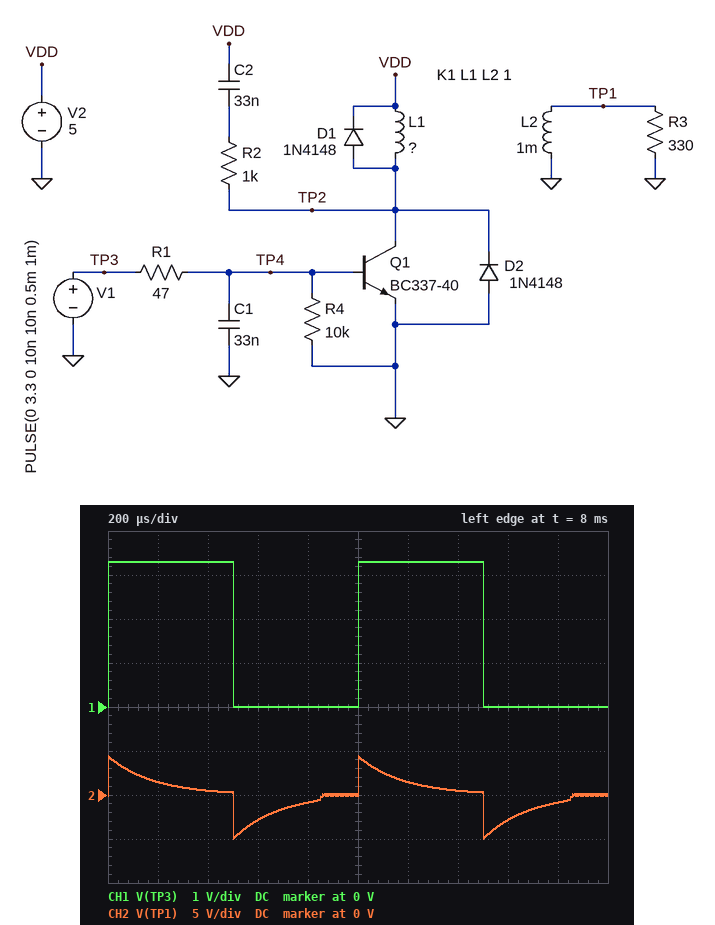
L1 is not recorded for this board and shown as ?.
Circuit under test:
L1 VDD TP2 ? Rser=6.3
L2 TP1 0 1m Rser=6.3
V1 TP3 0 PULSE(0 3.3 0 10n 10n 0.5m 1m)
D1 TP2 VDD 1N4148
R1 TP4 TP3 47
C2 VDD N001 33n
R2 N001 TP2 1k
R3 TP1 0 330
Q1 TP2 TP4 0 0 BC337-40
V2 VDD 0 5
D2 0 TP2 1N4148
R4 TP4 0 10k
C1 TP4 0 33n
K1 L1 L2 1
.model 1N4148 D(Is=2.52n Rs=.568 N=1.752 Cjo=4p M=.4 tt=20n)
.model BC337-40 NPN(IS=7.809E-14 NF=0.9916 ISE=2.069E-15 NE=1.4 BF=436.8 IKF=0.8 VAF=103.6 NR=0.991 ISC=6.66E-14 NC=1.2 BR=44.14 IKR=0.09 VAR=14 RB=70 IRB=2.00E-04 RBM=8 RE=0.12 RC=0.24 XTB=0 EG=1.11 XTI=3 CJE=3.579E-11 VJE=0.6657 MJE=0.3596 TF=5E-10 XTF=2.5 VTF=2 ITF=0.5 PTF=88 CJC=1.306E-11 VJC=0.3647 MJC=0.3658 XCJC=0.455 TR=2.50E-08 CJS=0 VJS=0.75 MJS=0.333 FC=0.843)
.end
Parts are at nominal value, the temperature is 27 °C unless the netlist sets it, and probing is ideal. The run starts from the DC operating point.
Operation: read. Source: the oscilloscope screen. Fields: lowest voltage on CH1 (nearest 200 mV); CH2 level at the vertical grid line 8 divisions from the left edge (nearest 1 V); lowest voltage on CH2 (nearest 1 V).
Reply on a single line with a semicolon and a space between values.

0 V; -3 V; -5 V
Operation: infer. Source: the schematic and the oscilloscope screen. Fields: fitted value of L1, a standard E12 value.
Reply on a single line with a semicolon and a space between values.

1.2 mH
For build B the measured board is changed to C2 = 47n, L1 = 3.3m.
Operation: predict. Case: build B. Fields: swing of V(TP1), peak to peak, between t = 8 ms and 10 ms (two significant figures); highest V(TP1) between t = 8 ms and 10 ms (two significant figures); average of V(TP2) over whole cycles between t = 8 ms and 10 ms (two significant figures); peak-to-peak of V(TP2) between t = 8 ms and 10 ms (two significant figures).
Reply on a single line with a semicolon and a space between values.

4.6 V; 2.3 V; 3.1 V; 6.1 V
